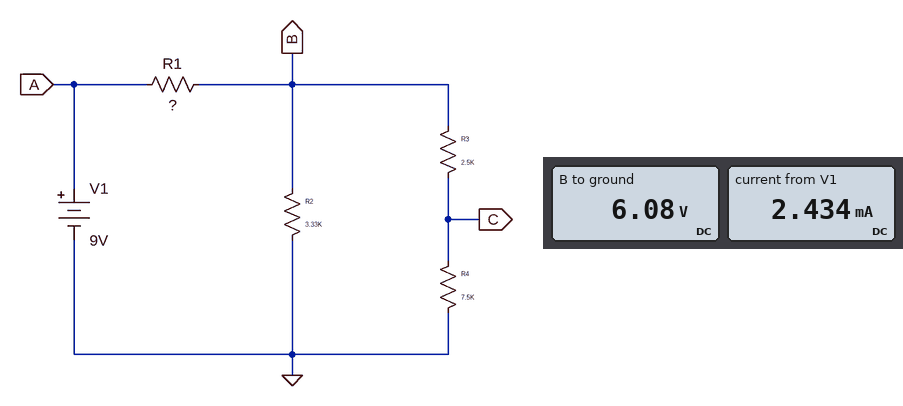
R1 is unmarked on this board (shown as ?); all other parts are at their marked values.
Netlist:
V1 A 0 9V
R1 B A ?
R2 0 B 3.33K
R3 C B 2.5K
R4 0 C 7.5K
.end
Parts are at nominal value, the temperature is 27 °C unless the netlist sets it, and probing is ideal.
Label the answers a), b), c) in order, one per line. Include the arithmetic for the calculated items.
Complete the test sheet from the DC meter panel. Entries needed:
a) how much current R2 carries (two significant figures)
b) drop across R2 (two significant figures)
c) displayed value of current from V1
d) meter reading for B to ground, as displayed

a) (6.08 V) / 3.33 kΩ = 1.8 mA
b) 6.08 V = 6.1 V
c) 2.434 mA
d) 6.08 V
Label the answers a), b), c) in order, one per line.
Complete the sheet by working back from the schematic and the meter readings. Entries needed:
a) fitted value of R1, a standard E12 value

a) 1.2 kΩ
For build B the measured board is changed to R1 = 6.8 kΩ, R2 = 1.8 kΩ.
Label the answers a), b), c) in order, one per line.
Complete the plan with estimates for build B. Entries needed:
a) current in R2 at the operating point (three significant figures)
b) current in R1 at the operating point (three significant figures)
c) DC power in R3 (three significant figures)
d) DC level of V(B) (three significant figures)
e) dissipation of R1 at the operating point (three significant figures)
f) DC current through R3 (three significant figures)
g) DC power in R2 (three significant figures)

a) 916 µA
b) 1.08 mA
c) 68.0 µW
d) 1.65 V
e) 7.95 mW
f) 165 µA
g) 1.51 mW
